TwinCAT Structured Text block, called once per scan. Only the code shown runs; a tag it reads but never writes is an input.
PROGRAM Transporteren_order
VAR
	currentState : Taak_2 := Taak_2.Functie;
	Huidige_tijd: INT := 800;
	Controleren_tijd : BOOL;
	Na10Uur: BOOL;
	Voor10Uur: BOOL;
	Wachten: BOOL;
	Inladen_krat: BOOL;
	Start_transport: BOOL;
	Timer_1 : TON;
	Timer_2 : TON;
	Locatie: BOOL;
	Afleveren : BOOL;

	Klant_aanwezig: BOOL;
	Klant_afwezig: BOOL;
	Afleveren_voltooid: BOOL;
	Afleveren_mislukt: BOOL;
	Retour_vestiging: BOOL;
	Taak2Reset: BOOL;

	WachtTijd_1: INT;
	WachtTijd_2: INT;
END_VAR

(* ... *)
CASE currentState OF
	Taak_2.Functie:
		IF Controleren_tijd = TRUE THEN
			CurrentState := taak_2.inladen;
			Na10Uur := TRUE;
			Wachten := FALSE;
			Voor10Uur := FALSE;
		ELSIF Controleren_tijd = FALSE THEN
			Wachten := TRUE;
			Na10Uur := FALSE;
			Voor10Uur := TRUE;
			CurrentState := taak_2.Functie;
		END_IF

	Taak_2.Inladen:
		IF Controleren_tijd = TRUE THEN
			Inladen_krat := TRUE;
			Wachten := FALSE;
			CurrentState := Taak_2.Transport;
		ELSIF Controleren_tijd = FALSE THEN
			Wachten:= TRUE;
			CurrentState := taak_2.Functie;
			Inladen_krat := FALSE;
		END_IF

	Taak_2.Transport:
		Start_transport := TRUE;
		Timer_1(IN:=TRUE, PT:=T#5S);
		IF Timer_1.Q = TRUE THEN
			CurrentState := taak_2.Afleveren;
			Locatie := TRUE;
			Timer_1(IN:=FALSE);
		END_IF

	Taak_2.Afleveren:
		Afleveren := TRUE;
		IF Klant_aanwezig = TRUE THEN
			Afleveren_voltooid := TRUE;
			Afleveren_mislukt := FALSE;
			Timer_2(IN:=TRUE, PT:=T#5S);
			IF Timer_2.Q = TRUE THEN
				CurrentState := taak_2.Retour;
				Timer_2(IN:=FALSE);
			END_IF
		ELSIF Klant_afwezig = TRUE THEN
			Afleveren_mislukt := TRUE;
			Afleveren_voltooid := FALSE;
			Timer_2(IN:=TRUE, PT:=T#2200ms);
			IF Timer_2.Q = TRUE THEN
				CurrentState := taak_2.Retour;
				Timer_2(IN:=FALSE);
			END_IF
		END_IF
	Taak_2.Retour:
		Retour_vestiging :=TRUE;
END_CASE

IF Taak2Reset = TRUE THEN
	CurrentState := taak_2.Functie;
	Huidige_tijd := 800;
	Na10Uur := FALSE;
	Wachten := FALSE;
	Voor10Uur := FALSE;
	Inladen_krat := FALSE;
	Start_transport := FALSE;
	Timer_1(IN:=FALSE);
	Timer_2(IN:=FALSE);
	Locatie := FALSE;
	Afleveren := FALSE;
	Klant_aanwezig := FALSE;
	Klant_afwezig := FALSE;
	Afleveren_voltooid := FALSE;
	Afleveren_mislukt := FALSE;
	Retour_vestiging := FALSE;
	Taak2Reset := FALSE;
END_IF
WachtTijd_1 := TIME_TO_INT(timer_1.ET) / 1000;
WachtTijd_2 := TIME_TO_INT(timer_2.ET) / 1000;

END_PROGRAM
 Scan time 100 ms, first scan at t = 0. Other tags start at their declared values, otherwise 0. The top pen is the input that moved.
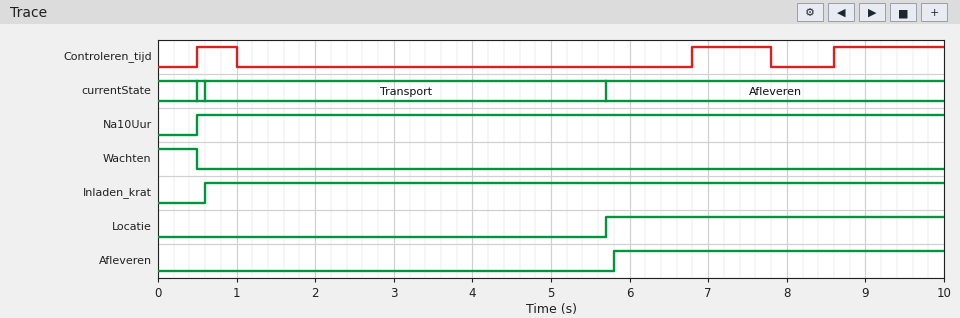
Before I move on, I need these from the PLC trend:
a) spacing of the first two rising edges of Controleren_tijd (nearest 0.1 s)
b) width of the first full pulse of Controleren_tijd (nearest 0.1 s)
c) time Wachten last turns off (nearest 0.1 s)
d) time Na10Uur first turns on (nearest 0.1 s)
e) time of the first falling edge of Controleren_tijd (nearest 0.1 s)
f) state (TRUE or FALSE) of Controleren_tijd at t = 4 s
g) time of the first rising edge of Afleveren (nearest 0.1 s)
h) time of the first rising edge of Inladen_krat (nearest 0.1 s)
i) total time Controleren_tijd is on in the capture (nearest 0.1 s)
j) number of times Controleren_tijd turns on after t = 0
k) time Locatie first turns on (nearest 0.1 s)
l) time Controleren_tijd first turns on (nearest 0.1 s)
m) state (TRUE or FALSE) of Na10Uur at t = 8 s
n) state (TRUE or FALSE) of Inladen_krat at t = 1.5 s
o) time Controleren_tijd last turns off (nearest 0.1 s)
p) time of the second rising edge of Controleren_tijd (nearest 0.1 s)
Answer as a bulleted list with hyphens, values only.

- 6.3 s
- 0.5 s
- 0.5 s
- 0.5 s
- 1.0 s
- FALSE
- 5.8 s
- 0.6 s
- 2.9 s
- 3
- 5.7 s
- 0.5 s
- TRUE
- TRUE
- 7.8 s
- 6.8 s
